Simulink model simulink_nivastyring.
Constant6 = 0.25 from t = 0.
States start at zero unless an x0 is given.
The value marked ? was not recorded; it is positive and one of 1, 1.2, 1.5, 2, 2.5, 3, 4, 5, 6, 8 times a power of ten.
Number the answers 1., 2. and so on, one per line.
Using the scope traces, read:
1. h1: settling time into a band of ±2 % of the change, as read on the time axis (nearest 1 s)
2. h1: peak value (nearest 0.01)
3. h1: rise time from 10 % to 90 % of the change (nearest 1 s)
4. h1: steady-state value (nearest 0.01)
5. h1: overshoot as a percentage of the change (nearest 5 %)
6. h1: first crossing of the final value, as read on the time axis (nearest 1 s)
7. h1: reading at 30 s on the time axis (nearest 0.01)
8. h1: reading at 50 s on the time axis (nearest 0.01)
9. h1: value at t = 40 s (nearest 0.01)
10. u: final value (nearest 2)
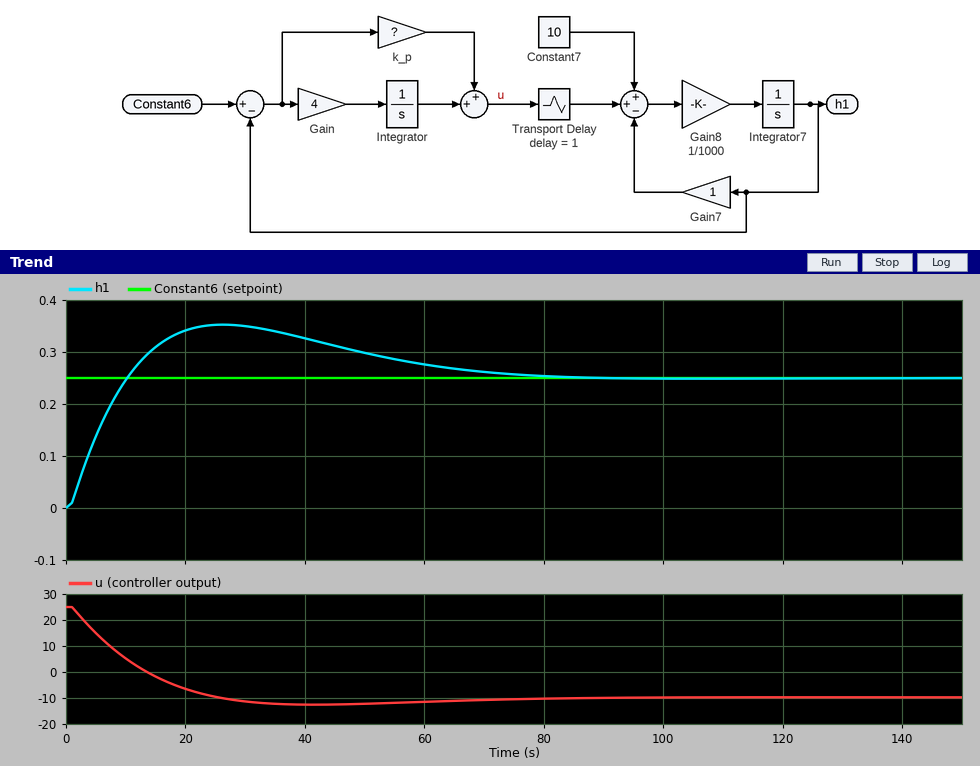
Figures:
1. 78 s
2. 0.35
3. 7 s
4. 0.25
5. 40 %
6. 10 s
7. 0.35
8. 0.30
9. 0.33
10. -10
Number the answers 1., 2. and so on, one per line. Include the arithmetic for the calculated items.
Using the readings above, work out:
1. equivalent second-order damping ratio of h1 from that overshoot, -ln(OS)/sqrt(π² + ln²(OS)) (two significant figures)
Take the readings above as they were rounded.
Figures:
1. ln(0.4) = -0.916; 0.916 / sqrt(9.870 + 0.840) = 0.28
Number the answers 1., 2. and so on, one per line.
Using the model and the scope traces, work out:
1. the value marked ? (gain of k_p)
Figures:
1. 100
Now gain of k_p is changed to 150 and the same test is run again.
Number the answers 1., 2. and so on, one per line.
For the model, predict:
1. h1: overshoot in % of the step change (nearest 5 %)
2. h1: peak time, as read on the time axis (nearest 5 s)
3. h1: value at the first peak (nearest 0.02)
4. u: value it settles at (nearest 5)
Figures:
1. 30 %
2. 20 s
3. 0.32
4. -10
